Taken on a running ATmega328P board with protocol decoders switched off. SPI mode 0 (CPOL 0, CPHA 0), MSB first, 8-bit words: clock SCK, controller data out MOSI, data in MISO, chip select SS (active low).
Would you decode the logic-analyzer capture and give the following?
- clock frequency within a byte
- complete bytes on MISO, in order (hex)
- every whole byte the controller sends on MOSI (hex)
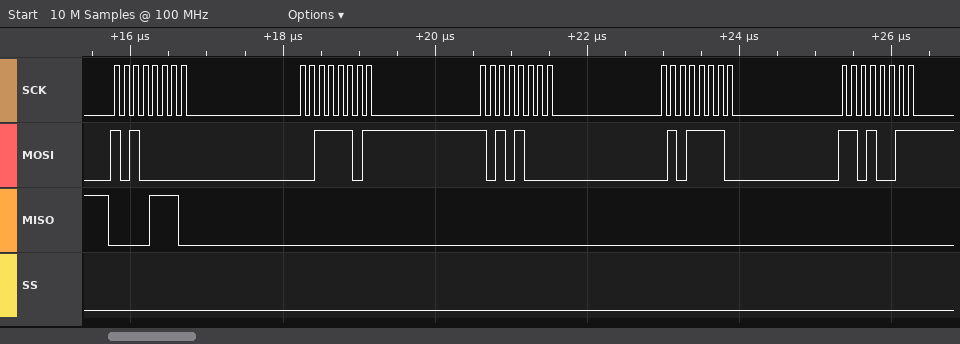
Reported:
8 MHz
0E 00 00 00 00
A0 3D A8 5E D3
